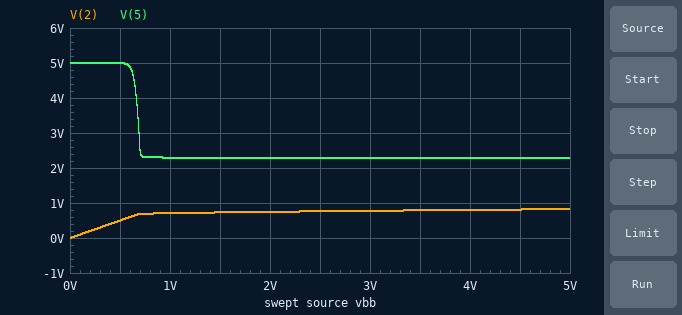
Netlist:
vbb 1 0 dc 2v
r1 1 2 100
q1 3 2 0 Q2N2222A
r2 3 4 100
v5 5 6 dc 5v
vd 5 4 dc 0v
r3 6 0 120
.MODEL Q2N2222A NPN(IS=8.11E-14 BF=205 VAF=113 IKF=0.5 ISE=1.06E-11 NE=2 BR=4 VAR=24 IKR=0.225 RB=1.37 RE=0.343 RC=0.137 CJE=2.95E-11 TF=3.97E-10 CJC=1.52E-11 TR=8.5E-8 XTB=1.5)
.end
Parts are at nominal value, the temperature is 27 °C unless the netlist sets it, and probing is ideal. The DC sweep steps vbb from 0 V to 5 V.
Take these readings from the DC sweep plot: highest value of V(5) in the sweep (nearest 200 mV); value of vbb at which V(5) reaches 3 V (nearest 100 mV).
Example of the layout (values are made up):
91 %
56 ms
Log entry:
5.0 V
700 mV
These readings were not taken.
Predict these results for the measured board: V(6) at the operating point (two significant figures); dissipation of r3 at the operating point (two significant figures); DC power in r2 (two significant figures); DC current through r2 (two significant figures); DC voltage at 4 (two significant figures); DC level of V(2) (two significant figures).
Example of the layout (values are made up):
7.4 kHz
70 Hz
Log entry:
-2.7 V
61 mW
51 mW
23 mA
2.3 V
750 mV
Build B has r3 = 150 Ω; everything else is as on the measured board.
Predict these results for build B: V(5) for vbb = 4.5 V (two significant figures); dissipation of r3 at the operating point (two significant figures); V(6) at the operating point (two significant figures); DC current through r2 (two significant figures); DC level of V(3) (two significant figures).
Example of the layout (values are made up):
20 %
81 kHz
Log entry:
2.0 V
59 mW
-3.0 V
20 mA
30 mV
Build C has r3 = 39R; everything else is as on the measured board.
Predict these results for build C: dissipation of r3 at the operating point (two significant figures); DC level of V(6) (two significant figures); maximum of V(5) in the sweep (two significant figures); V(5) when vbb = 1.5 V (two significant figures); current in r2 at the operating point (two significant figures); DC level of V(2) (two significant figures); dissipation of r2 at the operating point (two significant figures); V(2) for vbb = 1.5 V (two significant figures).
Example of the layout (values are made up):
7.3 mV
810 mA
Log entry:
50 mW
-1.4 V
5.0 V
3.6 V
36 mA
760 mV
130 mW
740 mV
